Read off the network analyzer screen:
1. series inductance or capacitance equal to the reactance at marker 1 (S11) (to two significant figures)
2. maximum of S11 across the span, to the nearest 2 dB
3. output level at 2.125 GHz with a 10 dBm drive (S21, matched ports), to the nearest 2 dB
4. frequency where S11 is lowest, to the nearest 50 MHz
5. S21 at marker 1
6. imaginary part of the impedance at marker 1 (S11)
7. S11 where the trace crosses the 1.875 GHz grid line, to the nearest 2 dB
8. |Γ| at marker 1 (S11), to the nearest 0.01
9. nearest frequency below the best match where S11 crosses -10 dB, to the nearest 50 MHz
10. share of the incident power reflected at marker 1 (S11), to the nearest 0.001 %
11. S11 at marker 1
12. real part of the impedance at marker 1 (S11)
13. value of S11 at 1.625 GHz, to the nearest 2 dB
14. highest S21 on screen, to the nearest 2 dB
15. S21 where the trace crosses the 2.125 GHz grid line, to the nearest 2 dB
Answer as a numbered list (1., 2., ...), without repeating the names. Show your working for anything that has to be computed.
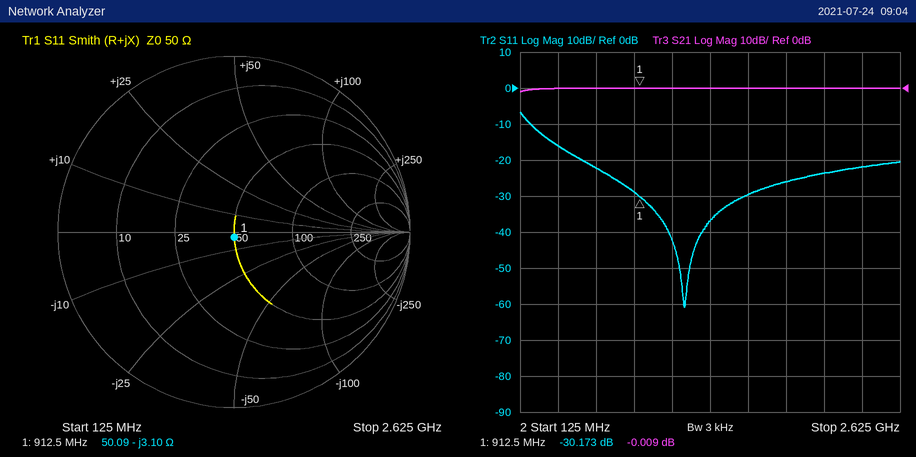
1. C = 1/(2π × 912.5 MHz × 3.1 Ω) ≈ 56 pF
2. -6 dB
3. 10 dBm + (0 dB) = 10 dBm
4. 1.20 GHz
5. -0.009 dB
6. -3.10 Ω
7. -26 dB
8. 0.03
9. 200 MHz
10. 10^(-30.173/10) ≈ 0.096 %
11. -30.173 dB
12. 50.09 Ω
13. -30 dB
14. 0 dB
15. 0 dB
